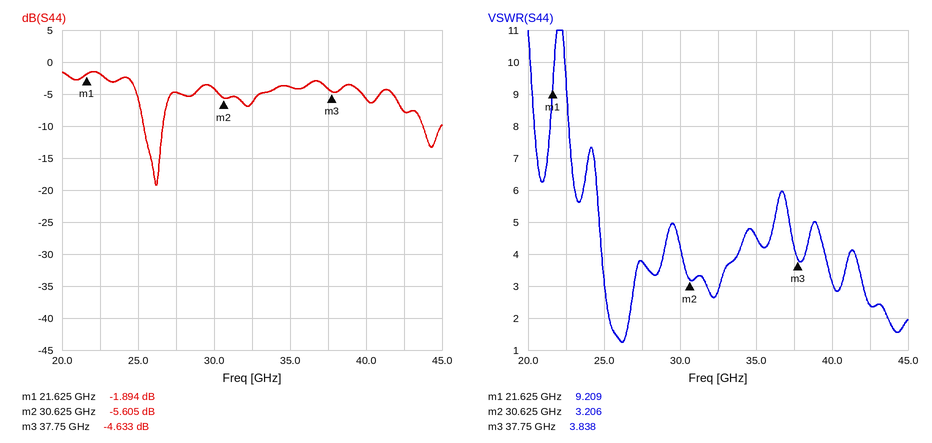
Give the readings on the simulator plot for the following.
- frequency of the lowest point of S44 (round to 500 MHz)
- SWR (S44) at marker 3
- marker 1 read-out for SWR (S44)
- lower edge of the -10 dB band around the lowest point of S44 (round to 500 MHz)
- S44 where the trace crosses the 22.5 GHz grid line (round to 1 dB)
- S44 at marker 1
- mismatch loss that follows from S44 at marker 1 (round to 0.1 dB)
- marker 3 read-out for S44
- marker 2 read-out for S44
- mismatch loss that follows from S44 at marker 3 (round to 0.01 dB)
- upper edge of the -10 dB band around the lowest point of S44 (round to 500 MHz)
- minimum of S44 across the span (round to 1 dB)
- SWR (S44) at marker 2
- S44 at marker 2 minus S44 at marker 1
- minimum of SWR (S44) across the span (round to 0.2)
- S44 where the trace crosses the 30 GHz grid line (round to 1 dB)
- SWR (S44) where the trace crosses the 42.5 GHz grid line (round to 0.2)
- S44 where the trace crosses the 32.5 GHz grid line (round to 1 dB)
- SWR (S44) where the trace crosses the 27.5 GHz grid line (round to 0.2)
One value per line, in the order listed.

26.0 GHz
3.838
9.209
25.5 GHz
-2 dB
-1.894 dB
4.5 dB
-4.633 dB
-5.605 dB
1.83 dB
26.5 GHz
-19 dB
3.206
-3.711 dB
1.2
-4 dB
2.4
-6 dB
3.8
